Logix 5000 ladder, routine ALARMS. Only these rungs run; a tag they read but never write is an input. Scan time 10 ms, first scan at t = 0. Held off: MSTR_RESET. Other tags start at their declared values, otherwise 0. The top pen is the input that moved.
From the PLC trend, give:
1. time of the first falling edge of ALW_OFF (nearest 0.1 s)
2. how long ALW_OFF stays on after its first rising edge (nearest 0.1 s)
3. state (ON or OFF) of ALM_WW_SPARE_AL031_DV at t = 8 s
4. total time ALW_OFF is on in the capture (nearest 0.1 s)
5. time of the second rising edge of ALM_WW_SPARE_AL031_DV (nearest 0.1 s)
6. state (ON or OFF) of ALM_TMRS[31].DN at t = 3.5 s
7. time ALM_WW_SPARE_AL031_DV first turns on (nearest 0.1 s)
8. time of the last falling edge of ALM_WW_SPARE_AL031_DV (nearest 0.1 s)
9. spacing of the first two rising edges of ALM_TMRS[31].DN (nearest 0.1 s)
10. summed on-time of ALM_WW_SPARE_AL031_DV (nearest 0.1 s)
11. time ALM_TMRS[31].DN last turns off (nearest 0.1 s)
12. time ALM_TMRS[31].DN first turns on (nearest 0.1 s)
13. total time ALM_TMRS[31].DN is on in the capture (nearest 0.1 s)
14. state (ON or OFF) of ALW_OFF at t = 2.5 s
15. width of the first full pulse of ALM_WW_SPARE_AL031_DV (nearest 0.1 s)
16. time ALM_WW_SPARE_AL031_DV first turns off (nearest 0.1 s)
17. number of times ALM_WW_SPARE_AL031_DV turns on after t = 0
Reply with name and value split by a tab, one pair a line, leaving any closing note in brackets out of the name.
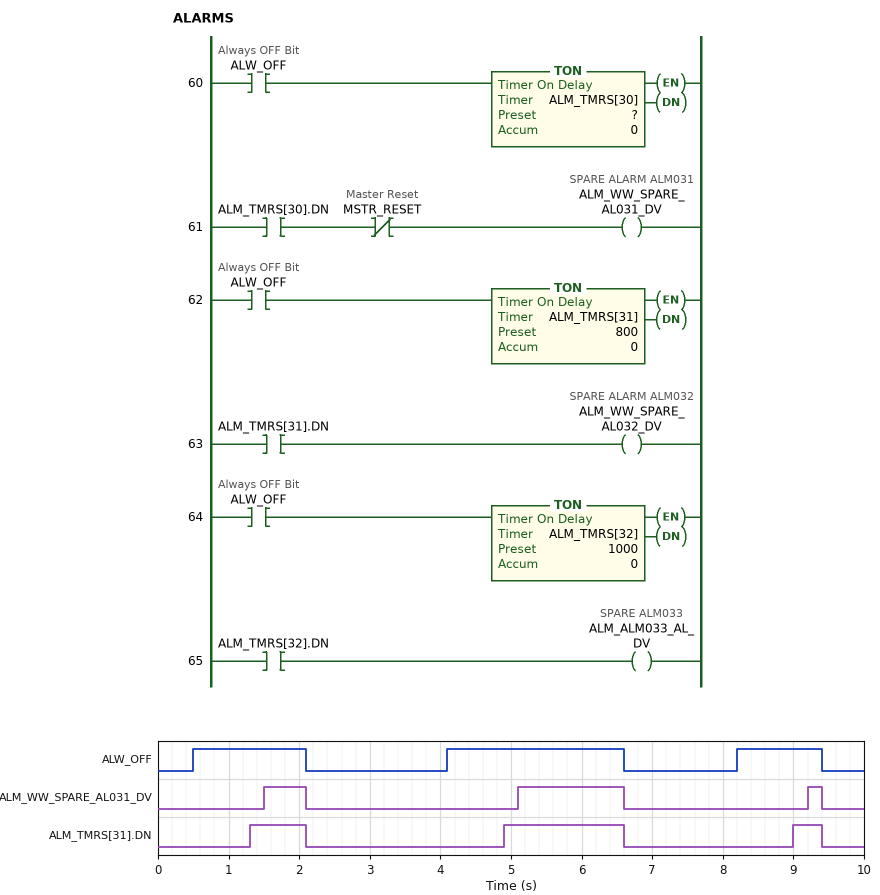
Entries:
time of the first falling edge of ALW_OFF	2.1 s
how long ALW_OFF stays on after its first rising edge	1.6 s
state (ON or OFF) of ALM_WW_SPARE_AL031_DV at t = 8 s	OFF
total time ALW_OFF is on in the capture	5.3 s
time of the second rising edge of ALM_WW_SPARE_AL031_DV	5.1 s
state (ON or OFF) of ALM_TMRS[31].DN at t = 3.5 s	OFF
time ALM_WW_SPARE_AL031_DV first turns on	1.5 s
time of the last falling edge of ALM_WW_SPARE_AL031_DV	9.4 s
spacing of the first two rising edges of ALM_TMRS[31].DN	3.6 s
summed on-time of ALM_WW_SPARE_AL031_DV	2.3 s
time ALM_TMRS[31].DN last turns off	9.4 s
time ALM_TMRS[31].DN first turns on	1.3 s
total time ALM_TMRS[31].DN is on in the capture	2.9 s
state (ON or OFF) of ALW_OFF at t = 2.5 s	OFF
width of the first full pulse of ALM_WW_SPARE_AL031_DV	0.6 s
time ALM_WW_SPARE_AL031_DV first turns off	2.1 s
number of times ALM_WW_SPARE_AL031_DV turns on after t = 0	3
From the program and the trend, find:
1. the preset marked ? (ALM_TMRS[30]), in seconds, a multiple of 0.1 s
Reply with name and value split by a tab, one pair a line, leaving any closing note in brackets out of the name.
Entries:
the preset marked ? (ALM_TMRS[30]), in seconds, a multiple of 0.1 s	1.0 s
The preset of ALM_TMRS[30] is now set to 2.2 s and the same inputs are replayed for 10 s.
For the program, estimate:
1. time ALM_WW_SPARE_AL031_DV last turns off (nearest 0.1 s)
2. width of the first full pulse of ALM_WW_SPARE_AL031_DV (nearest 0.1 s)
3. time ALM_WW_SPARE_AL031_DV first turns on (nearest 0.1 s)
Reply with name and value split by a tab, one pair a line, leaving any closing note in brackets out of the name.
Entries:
time ALM_WW_SPARE_AL031_DV last turns off	6.6 s
width of the first full pulse of ALM_WW_SPARE_AL031_DV	0.3 s
time ALM_WW_SPARE_AL031_DV first turns on	6.3 s
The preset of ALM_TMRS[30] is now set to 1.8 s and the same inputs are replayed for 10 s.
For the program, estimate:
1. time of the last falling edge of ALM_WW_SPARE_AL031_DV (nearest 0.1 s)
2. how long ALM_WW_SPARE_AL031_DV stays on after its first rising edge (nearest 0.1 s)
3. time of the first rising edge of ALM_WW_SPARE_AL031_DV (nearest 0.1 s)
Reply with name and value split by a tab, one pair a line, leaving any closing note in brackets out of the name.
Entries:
time of the last falling edge of ALM_WW_SPARE_AL031_DV	6.6 s
how long ALM_WW_SPARE_AL031_DV stays on after its first rising edge	0.7 s
time of the first rising edge of ALM_WW_SPARE_AL031_DV	5.9 s
